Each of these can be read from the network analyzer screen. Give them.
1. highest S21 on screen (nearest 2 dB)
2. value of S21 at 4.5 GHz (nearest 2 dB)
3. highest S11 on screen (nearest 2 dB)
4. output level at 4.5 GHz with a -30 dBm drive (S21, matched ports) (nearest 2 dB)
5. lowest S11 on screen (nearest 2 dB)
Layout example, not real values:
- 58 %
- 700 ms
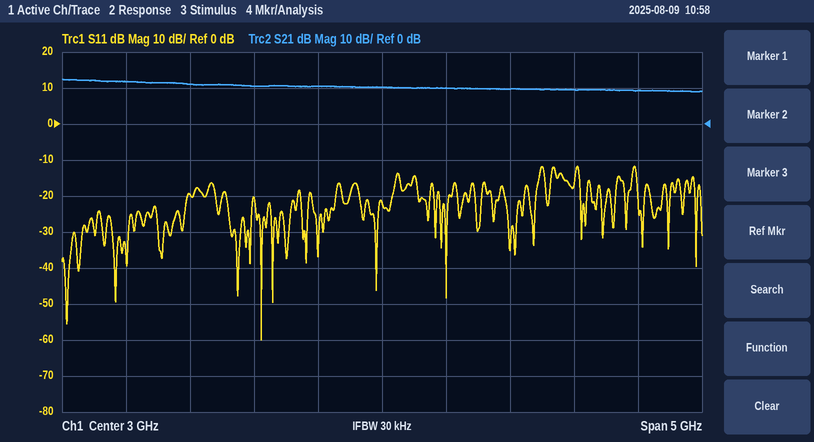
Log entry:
- 12 dB
- 10 dB
- -12 dB
- -20 dBm
- -60 dB
